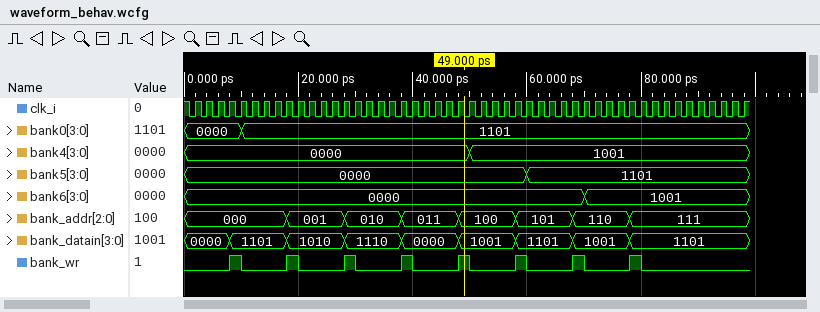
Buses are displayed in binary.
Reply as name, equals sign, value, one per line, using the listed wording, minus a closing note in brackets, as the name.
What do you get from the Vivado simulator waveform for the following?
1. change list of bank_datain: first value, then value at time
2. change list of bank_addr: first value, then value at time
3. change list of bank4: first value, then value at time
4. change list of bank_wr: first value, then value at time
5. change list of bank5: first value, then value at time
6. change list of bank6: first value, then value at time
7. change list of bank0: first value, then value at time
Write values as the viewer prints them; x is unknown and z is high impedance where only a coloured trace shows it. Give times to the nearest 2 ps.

change list of bank_datain: first value, then value at time = 0000, 1101 at 8 ps, 1010 at 18 ps, 1110 at 28 ps, 0000 at 38 ps, 1001 at 48 ps, 1101 at 58 ps, 1001 at 68 ps, 1101 at 78 ps
change list of bank_addr: first value, then value at time = 000, 001 at 18 ps, 010 at 28 ps, 011 at 38 ps, 100 at 48 ps, 101 at 58 ps, 110 at 68 ps, 111 at 78 ps
change list of bank4: first value, then value at time = 0000, 1001 at 50 ps
change list of bank_wr: first value, then value at time = 0, 1 at 8 ps, 0 at 10 ps, 1 at 18 ps, 0 at 20 ps, 1 at 28 ps, 0 at 30 ps, 1 at 38 ps, 0 at 40 ps, 1 at 48 ps, 0 at 50 ps, 1 at 58 ps, 0 at 60 ps, 1 at 68 ps, 0 at 70 ps, 1 at 78 ps, 0 at 80 ps
change list of bank5: first value, then value at time = 0000, 1101 at 60 ps
change list of bank6: first value, then value at time = 0000, 1001 at 70 ps
change list of bank0: first value, then value at time = 0000, 1101 at 10 ps
